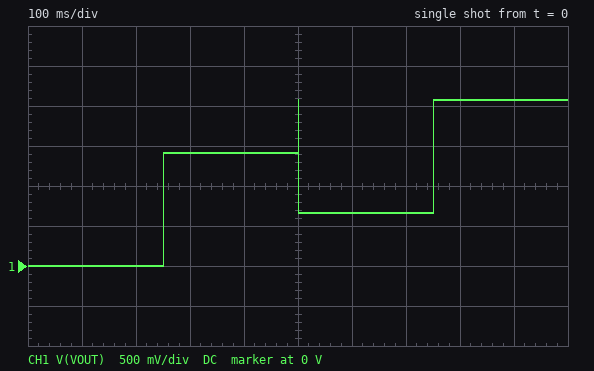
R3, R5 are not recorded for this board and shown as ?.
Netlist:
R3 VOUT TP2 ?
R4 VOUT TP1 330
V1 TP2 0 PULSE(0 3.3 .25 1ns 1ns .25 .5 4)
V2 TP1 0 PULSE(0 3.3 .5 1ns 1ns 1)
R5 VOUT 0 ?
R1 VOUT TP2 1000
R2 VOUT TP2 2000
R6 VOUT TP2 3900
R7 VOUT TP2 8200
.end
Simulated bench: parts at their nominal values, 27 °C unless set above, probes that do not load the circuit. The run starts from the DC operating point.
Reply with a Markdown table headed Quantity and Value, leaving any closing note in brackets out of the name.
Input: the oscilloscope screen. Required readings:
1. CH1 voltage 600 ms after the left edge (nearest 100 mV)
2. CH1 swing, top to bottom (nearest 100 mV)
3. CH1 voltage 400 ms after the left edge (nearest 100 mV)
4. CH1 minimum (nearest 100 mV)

| Quantity | Value |
|---|---|
| CH1 voltage 600 ms after the left edge | 700 mV |
| CH1 swing, top to bottom | 2.1 V |
| CH1 voltage 400 ms after the left edge | 1.4 V |
| CH1 minimum | 0 V |
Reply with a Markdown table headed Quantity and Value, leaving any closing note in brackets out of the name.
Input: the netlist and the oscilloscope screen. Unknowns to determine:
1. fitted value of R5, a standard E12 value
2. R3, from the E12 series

| Quantity | Value |
|---|---|
| fitted value of R5, a standard E12 value | 180 Ω |
| R3, from the E12 series | 220 Ω |
